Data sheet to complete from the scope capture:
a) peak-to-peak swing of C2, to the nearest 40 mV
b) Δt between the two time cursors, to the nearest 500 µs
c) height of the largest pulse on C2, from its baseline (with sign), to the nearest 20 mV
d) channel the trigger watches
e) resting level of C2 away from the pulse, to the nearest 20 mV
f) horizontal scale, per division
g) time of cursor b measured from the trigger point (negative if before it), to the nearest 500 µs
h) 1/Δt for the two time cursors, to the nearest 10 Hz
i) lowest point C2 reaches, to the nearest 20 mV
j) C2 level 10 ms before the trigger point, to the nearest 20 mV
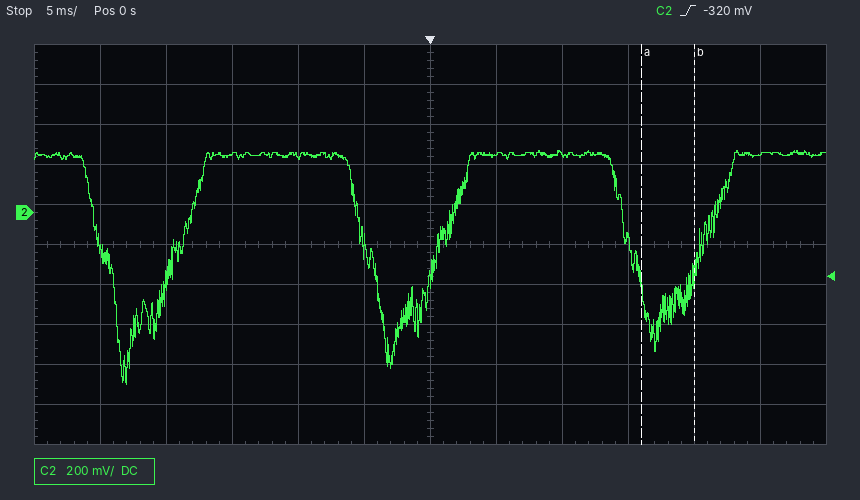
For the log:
1.16 V
4.0 ms
-1.14 V
C2
280 mV
5 ms
+20.0 ms
250 Hz
-860 mV
280 mV
